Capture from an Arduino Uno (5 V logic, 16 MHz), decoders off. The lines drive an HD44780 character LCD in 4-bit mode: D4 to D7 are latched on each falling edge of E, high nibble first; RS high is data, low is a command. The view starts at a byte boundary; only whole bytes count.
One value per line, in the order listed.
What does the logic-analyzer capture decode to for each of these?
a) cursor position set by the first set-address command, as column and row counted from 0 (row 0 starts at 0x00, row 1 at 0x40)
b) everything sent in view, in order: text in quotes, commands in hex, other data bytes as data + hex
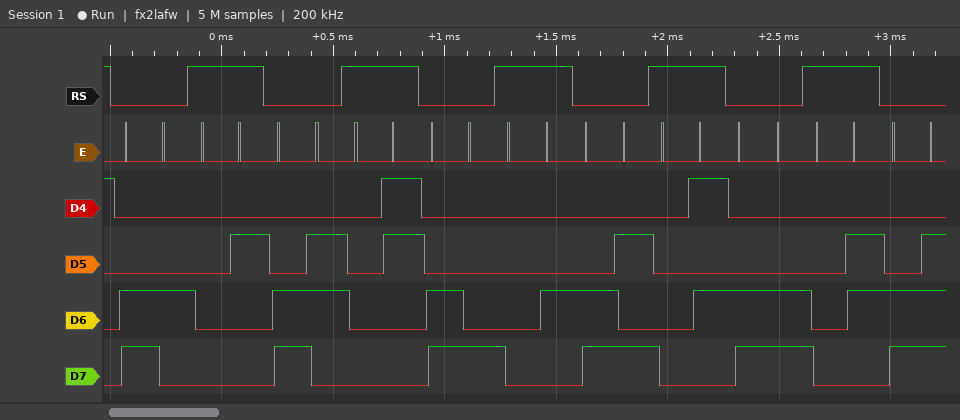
column 4, row 1
0xC4 data 02 0xC6 data 03 0xC8 data 04 0xCA data 05 0xCC data 06 0xCE
